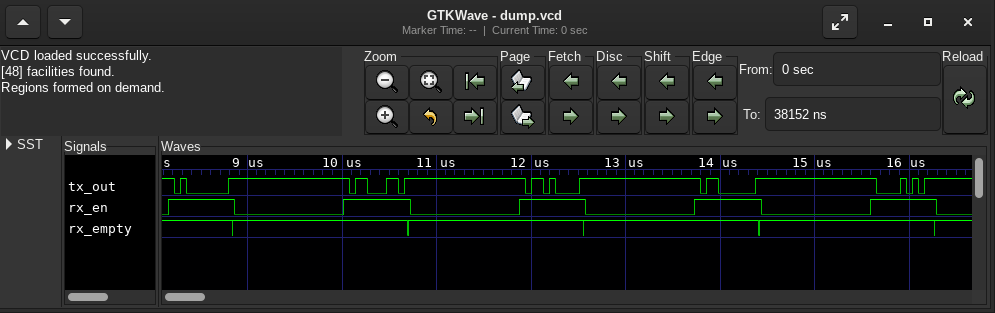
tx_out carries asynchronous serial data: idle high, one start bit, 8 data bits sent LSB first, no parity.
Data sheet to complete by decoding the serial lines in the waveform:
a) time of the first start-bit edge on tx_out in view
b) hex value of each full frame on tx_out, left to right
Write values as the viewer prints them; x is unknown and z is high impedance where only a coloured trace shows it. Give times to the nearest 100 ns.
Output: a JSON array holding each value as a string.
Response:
["8200 ns", "01, 63, 0B, 03, A8"]
